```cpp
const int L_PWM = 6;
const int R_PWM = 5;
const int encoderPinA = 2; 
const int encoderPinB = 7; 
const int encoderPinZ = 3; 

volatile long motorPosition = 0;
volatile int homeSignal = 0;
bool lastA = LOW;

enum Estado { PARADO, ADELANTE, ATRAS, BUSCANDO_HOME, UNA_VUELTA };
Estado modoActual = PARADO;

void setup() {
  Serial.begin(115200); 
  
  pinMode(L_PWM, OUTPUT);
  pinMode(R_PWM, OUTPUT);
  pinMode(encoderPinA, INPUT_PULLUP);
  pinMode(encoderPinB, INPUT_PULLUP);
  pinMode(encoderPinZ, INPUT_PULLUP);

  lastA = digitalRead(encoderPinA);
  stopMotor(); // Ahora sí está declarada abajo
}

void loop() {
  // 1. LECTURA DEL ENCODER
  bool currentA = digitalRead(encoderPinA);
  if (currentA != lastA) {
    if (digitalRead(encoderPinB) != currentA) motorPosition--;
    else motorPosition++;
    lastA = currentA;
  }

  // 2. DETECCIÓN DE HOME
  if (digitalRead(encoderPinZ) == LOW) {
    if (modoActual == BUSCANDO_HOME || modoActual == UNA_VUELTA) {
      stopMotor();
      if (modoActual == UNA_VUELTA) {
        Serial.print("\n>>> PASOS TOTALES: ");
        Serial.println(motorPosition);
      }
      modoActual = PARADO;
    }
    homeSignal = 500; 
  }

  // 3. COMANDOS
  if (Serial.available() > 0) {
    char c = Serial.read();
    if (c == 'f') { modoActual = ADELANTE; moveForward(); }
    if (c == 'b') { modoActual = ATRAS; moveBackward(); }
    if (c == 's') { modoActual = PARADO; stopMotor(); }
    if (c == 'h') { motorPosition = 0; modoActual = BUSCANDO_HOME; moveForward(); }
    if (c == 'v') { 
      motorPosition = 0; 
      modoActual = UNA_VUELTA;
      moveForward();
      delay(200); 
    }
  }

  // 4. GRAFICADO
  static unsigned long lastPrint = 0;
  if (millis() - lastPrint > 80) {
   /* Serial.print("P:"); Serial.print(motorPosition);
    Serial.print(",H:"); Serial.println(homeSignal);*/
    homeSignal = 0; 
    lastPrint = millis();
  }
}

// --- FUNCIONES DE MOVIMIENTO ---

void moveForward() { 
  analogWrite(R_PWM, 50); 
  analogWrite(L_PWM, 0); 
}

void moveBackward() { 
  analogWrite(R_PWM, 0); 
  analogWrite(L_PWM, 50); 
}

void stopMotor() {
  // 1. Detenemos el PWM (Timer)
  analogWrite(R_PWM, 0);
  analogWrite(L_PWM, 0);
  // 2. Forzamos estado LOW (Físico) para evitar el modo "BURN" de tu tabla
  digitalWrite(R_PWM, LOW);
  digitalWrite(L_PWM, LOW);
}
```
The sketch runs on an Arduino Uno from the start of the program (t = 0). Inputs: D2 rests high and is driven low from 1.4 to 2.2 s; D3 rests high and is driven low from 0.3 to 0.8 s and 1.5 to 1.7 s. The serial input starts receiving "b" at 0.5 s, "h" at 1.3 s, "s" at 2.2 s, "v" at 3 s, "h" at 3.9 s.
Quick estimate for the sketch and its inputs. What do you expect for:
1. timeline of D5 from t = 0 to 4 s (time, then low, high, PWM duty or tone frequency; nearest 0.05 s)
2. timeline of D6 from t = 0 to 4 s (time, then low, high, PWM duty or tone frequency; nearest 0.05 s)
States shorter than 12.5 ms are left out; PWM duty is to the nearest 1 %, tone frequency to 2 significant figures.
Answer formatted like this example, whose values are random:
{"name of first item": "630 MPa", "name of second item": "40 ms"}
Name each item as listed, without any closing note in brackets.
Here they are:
{"timeline of D5 from t = 0 to 4 s": "0 s low; 1.3 s PWM 20 %; 1.5 s low; 3 s PWM 20 %", "timeline of D6 from t = 0 to 4 s": "0 s low; 0.5 s PWM 20 %; 1.3 s low"}
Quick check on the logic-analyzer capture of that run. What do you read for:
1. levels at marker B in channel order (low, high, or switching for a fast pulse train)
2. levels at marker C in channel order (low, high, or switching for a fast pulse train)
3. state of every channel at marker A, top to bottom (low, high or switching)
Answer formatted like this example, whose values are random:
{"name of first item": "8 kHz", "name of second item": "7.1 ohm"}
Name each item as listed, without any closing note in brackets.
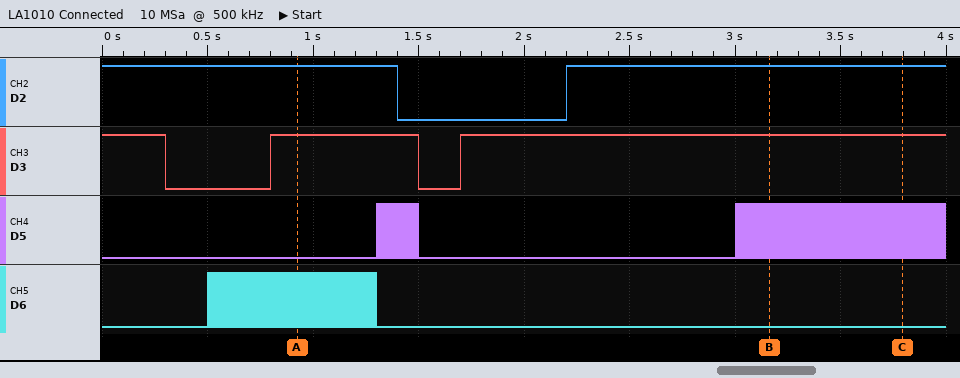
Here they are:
{"levels at marker B in channel order": "D2 high, D3 high, D5 switching, D6 low", "levels at marker C in channel order": "D2 high, D3 high, D5 switching, D6 low", "state of every channel at marker A, top to bottom": "D2 high, D3 high, D5 low, D6 switching"}
